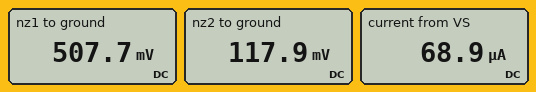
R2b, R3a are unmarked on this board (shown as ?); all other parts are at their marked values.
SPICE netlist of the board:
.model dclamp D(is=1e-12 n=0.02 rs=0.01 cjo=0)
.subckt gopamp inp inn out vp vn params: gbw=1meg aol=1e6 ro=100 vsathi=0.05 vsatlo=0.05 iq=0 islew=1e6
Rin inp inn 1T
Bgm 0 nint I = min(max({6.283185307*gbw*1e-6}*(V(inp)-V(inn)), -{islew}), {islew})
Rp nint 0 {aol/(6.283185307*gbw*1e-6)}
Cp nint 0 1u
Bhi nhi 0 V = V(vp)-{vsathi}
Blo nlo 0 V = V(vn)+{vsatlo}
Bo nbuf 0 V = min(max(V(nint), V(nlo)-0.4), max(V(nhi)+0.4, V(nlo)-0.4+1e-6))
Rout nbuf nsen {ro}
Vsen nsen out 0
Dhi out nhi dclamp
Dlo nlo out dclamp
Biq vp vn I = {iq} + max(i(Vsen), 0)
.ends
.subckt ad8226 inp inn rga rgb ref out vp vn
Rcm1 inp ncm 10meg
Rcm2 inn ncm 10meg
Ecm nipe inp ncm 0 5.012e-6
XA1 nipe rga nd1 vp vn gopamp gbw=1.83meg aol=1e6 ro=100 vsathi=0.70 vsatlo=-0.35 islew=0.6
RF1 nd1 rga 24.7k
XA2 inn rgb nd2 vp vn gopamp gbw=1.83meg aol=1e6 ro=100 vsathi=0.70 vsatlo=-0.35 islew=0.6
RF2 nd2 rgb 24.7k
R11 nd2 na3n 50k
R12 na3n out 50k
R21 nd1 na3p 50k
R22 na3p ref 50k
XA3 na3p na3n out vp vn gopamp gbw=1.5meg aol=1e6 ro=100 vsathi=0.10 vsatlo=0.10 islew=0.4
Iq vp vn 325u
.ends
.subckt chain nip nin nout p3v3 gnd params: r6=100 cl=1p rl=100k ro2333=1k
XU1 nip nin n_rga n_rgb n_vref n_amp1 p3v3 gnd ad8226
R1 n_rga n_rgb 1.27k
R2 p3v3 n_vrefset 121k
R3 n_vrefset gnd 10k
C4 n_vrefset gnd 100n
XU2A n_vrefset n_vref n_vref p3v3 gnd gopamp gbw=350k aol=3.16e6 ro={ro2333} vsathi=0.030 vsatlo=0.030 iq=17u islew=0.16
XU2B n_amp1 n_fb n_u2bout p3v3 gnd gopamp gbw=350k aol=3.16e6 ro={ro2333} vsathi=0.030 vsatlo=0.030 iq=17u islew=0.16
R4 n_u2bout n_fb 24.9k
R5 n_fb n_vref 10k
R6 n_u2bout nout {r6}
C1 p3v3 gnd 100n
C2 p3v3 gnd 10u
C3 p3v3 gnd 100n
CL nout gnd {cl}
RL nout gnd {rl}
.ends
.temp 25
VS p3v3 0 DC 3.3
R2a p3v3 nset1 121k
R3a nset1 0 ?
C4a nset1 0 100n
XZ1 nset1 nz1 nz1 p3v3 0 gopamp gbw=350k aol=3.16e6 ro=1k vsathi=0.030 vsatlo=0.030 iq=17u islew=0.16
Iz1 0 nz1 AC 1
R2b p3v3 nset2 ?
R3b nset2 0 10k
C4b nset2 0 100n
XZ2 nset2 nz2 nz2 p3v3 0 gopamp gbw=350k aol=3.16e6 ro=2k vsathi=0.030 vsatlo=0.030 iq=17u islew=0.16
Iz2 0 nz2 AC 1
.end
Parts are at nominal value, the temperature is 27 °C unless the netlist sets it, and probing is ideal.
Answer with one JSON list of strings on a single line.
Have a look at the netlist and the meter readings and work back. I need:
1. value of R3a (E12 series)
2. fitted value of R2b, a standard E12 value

["22 kΩ", "270 kΩ"]
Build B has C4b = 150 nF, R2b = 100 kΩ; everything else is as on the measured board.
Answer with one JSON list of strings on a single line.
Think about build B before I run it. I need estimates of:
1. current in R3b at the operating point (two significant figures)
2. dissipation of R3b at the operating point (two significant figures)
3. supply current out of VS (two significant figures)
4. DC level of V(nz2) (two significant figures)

["30 µA", "9.0 µW", "87 µA", "300 mV"]
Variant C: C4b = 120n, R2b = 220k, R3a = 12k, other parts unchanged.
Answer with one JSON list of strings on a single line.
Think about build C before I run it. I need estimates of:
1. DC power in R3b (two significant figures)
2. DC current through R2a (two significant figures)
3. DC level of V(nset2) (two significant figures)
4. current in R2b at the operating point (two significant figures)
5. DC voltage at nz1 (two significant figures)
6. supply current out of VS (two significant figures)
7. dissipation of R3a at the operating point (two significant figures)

["2.1 µW", "25 µA", "140 mV", "14 µA", "300 mV", "73 µA", "7.4 µW"]
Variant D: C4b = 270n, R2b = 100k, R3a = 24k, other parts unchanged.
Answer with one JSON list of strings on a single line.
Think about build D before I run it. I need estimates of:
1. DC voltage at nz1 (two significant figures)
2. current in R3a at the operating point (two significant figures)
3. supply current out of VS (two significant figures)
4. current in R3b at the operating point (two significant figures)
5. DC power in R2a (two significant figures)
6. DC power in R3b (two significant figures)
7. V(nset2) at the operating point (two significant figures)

["550 mV", "23 µA", "87 µA", "30 µA", "63 µW", "9.0 µW", "300 mV"]
